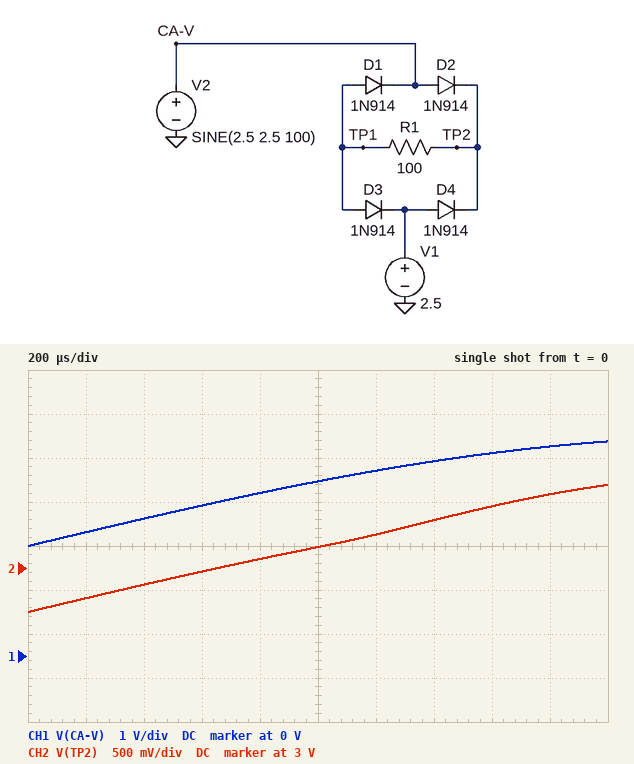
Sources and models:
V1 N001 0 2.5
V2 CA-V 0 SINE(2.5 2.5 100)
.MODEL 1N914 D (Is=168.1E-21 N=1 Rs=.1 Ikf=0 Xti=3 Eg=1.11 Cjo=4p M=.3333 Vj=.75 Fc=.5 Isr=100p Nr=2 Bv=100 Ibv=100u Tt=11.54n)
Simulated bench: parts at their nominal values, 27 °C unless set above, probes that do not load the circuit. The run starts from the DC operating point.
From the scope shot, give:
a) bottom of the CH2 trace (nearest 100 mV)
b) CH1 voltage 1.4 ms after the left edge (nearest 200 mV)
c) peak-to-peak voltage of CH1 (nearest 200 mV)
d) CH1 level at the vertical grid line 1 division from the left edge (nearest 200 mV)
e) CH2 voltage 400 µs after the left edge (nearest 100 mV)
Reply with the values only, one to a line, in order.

2.5 V
4.4 V
2.4 V
2.8 V
2.8 V
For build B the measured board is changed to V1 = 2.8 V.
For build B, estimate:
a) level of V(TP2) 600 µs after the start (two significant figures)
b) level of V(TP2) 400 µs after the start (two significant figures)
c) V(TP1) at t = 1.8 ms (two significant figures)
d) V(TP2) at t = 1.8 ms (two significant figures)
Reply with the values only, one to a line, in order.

3.1 V
3.0 V
3.7 V
3.9 V
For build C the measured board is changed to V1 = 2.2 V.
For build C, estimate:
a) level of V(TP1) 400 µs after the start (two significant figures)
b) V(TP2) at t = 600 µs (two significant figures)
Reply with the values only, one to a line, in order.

2.7 V
2.8 V
